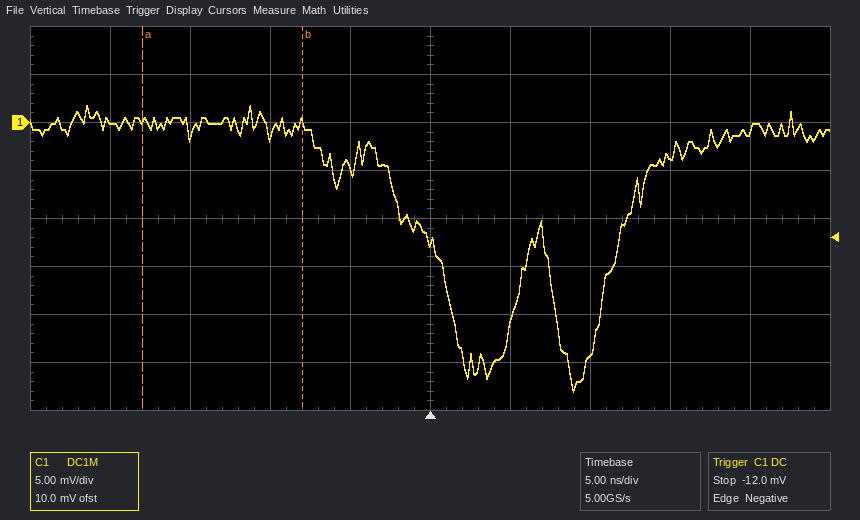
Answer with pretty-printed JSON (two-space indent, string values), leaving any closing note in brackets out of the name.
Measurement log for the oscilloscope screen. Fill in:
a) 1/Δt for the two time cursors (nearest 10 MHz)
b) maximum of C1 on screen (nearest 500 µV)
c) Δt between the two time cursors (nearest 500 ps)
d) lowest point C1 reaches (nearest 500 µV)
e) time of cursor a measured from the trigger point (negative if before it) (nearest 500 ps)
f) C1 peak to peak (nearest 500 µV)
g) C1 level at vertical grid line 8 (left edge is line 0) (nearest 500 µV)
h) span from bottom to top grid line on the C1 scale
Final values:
{
  "1/Δt for the two time cursors": "100 MHz",
  "maximum of C1 on screen": "2.0 mV",
  "Δt between the two time cursors": "10.0 ns",
  "lowest point C1 reaches": "-28.0 mV",
  "time of cursor a measured from the trigger point (negative if before it)": "-18.0 ns",
  "C1 peak to peak": "30.0 mV",
  "C1 level at vertical grid line 8 (left edge is line 0)": "-3.5 mV",
  "span from bottom to top grid line on the C1 scale": "40 mV"
}
